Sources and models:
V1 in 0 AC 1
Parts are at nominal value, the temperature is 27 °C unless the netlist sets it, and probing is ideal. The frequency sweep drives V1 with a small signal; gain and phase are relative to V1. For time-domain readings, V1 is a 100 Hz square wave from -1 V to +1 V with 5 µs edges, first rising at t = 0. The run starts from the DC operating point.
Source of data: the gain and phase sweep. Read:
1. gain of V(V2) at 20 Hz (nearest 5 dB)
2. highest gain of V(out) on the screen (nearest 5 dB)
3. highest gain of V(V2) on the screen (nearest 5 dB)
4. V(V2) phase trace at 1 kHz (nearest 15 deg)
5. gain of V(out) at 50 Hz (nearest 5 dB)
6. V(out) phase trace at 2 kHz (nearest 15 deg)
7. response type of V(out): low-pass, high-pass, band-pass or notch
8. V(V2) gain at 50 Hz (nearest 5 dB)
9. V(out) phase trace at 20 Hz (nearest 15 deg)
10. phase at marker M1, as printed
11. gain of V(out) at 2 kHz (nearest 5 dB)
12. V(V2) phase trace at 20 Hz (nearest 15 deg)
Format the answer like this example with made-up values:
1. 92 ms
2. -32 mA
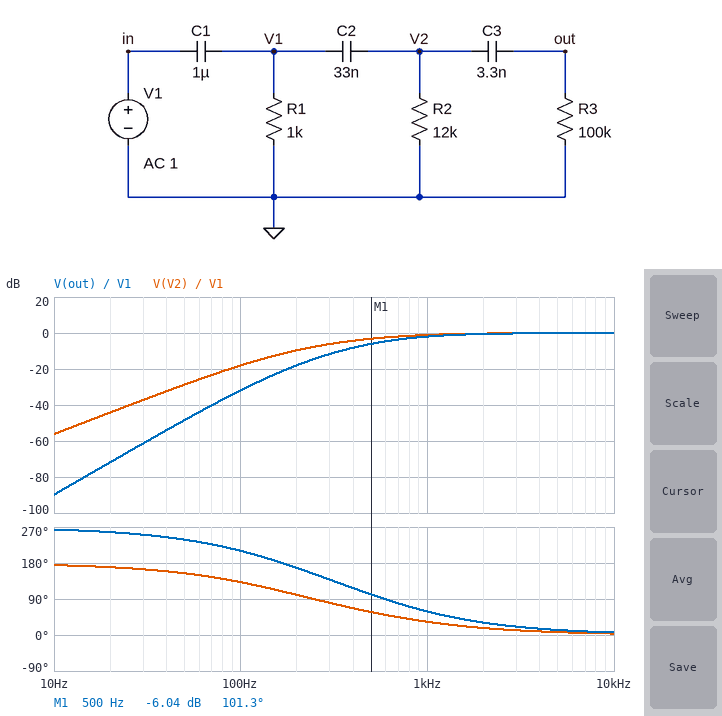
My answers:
1. -45 dB
2. 0 dB
3. 0 dB
4. 30 deg
5. -50 dB
6. 30 deg
7. high-pass
8. -30 dB
9. 255 deg
10. 101.3 deg
11. 0 dB
12. 165 deg
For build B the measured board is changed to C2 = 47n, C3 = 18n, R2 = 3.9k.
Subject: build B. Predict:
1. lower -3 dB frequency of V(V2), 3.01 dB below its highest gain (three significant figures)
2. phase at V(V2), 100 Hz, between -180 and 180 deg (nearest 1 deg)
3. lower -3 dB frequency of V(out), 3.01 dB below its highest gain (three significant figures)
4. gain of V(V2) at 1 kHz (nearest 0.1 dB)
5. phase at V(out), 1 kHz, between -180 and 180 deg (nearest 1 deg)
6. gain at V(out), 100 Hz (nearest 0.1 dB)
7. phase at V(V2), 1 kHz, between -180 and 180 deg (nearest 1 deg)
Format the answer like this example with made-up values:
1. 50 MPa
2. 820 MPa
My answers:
1. 979 Hz
2. 139 deg
3. 987 Hz
4. -2.9 dB
5. 57 deg
6. -27.2 dB
7. 52 deg
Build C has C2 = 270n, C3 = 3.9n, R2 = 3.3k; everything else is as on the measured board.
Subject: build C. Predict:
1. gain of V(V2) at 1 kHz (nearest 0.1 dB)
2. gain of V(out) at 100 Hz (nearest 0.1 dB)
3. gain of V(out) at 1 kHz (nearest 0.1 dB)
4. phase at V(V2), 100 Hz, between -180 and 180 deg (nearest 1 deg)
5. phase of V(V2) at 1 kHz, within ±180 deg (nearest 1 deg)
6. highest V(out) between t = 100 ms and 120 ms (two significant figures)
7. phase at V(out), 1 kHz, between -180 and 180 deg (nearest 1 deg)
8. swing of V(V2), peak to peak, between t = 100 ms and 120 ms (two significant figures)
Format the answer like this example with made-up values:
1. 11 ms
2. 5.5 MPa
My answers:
1. -0.4 dB
2. -25.1 dB
3. -1.1 dB
4. 115 deg
5. 22 deg
6. 2.0 V
7. 44 deg
8. 4.1 V
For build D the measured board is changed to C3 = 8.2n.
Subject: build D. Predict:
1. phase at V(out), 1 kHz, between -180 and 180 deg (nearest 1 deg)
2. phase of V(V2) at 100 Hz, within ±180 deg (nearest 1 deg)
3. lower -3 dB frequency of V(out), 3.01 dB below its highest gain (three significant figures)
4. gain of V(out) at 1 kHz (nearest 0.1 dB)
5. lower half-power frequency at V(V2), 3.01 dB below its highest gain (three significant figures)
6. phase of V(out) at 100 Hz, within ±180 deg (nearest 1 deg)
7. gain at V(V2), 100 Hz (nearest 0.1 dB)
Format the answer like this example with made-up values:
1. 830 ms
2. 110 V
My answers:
1. 45 deg
2. 131 deg
3. 586 Hz
4. -1.2 dB
5. 527 Hz
6. -166 deg
7. -18.2 dB
